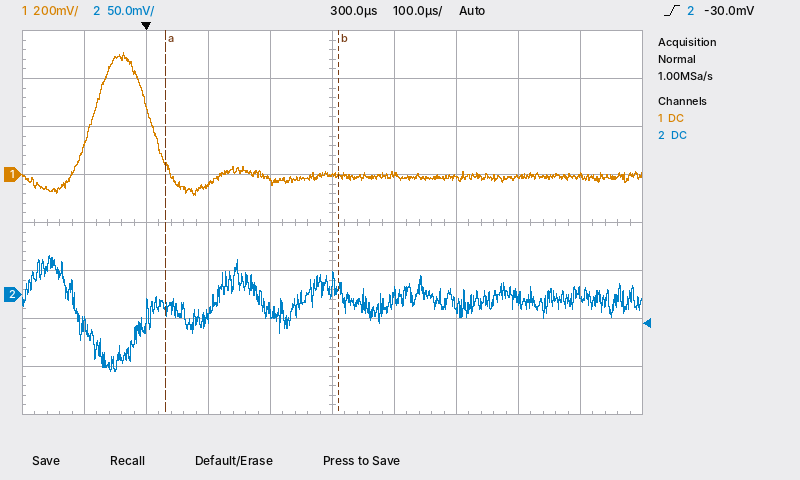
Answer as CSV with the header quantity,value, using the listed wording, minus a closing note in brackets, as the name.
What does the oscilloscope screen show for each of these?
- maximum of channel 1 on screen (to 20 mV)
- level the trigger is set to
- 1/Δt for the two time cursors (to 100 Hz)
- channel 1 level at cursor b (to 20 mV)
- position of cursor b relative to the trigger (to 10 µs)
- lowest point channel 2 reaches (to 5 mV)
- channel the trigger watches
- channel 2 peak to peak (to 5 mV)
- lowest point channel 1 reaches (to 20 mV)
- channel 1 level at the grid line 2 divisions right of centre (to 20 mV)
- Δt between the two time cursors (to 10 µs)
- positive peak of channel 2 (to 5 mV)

quantity,value
maximum of channel 1 on screen,500 mV
level the trigger is set to,-30.0 mV
1/Δt for the two time cursors,3.6 kHz
channel 1 level at cursor b,0 mV
position of cursor b relative to the trigger,+310 µs
lowest point channel 2 reaches,-80 mV
channel the trigger watches,channel 2
channel 2 peak to peak,120 mV
lowest point channel 1 reaches,-80 mV
channel 1 level at the grid line 2 divisions right of centre,-20 mV
Δt between the two time cursors,280 µs
positive peak of channel 2,40 mV
